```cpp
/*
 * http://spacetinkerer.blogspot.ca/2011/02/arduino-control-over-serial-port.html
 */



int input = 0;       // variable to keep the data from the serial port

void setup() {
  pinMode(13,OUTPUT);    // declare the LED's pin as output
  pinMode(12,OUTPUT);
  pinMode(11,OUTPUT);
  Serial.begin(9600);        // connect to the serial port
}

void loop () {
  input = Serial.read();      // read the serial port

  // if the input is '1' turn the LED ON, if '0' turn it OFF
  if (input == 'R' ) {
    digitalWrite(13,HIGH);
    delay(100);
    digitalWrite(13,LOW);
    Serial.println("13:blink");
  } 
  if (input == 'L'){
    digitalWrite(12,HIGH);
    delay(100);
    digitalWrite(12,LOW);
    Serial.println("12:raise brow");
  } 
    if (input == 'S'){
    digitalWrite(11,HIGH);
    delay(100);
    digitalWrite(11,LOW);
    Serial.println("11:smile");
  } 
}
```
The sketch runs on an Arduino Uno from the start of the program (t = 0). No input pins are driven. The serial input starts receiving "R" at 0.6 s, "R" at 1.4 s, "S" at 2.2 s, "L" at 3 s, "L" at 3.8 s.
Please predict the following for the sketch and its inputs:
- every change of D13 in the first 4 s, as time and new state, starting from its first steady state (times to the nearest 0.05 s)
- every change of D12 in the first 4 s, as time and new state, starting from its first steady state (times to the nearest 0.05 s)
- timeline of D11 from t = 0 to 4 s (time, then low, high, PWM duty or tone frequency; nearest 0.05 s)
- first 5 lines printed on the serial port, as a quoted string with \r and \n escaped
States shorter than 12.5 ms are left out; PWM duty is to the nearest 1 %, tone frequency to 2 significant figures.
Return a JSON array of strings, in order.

["0 s low; 0.6 s high; 0.7 s low; 1.4 s high; 1.5 s low", "0 s low; 3 s high; 3.1 s low; 3.8 s high; 3.9 s low", "0 s low; 2.2 s high; 2.3 s low", "\"13:blink\\r\\n13:blink\\r\\n11:smile\\r\\n12:raise brow\\r\\n12:raise brow\\r\\n\""]
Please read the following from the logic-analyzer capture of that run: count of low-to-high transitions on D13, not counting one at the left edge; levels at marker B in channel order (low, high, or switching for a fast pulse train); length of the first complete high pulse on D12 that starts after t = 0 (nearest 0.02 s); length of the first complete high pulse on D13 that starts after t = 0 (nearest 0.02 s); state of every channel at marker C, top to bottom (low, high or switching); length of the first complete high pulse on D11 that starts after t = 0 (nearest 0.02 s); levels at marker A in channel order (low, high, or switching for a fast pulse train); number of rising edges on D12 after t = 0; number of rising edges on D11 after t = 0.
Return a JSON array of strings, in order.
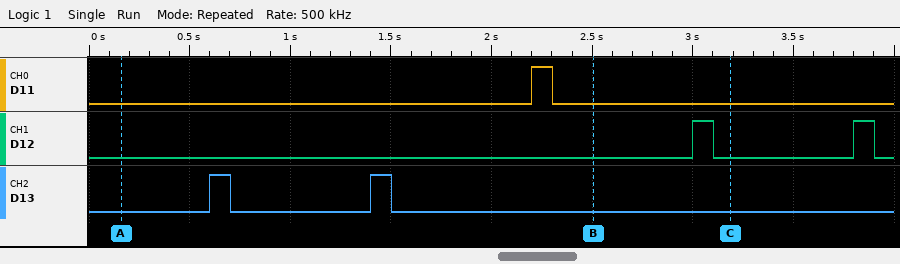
["2", "D11 low, D12 low, D13 low", "0.10 s", "0.10 s", "D11 low, D12 low, D13 low", "0.10 s", "D11 low, D12 low, D13 low", "2", "1"]
